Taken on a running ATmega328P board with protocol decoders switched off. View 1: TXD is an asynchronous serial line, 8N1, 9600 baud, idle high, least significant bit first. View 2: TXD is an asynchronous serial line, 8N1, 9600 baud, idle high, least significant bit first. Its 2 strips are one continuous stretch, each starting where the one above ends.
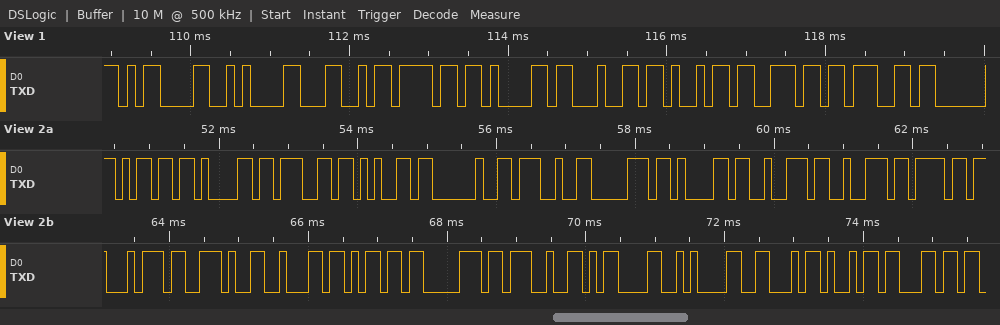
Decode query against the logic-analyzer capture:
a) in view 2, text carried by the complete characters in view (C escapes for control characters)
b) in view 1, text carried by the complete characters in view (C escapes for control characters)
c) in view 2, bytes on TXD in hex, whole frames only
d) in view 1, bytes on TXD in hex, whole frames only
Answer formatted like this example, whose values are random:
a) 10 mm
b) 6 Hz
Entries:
a) "mage 'parrot.bmp'\r\nFil"
b) "\r\nLoading"
c) 6D 61 67 65 20 27 70 61 72 72 6F 74 2E 62 6D 70 27 0D 0A 46 69 6C
d) 0D 0A 4C 6F 61 64 69 6E 67
